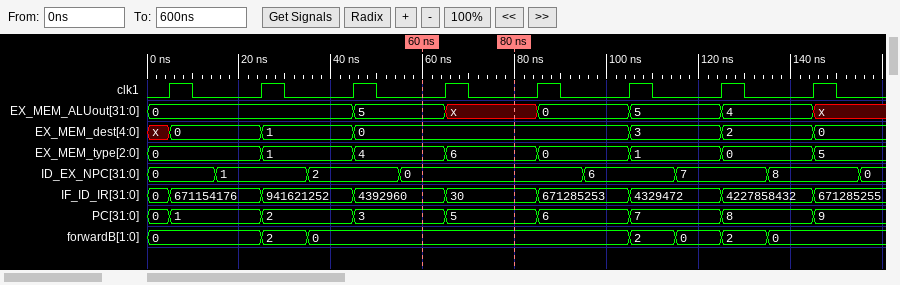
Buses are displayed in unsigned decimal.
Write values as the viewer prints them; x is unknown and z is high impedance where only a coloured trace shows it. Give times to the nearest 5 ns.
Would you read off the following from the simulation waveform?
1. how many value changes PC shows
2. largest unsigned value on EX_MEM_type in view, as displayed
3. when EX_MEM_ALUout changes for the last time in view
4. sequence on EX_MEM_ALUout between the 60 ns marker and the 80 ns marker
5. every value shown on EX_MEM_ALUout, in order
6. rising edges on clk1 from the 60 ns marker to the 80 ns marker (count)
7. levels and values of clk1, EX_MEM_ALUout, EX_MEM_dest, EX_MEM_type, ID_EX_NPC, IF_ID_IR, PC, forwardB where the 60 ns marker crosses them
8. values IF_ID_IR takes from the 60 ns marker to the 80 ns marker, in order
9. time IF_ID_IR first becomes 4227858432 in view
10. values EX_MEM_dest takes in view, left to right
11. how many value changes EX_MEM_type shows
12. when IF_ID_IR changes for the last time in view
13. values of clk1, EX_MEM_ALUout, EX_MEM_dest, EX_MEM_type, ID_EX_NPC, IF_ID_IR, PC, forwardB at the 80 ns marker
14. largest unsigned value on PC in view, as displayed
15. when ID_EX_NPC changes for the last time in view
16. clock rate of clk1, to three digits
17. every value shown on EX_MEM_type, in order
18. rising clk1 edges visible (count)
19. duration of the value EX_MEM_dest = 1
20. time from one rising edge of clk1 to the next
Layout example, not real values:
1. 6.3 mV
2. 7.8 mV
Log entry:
1. 8
2. 6
3. 145 ns
4. 5, x
5. 0, 5, x, 0, 5, 4, x
6. 1
7. clk1=0, EX_MEM_ALUout=5, EX_MEM_dest=0, EX_MEM_type=4, ID_EX_NPC=0, IF_ID_IR=4392960, PC=3, forwardB=0
8. 4392960, 30
9. 125 ns
10. x, 0, 1, 0, 3, 2, 0
11. 7
12. 145 ns
13. clk1=0, EX_MEM_ALUout=x, EX_MEM_dest=0, EX_MEM_type=6, ID_EX_NPC=0, IF_ID_IR=30, PC=5, forwardB=0
14. 9
15. 155 ns
16. 50.0 MHz
17. 0, 1, 4, 6, 0, 1, 0, 5
18. 8
19. 20 ns
20. 20 ns
